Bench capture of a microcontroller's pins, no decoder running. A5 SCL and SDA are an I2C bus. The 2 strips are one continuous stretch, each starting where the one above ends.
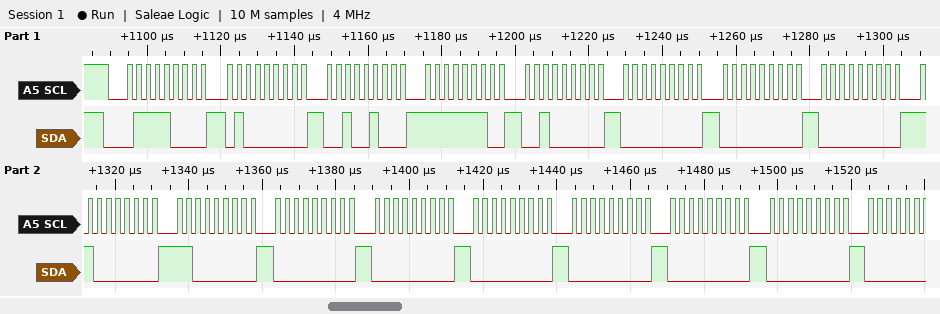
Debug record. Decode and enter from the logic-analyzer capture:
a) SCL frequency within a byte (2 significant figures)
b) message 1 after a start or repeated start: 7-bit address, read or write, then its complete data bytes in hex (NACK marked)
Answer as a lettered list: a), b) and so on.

a) 400 kHz
b) 0x3C write: 40 24 FE 20 00 00 00 C0 C0 00 00 00 00 00 00
